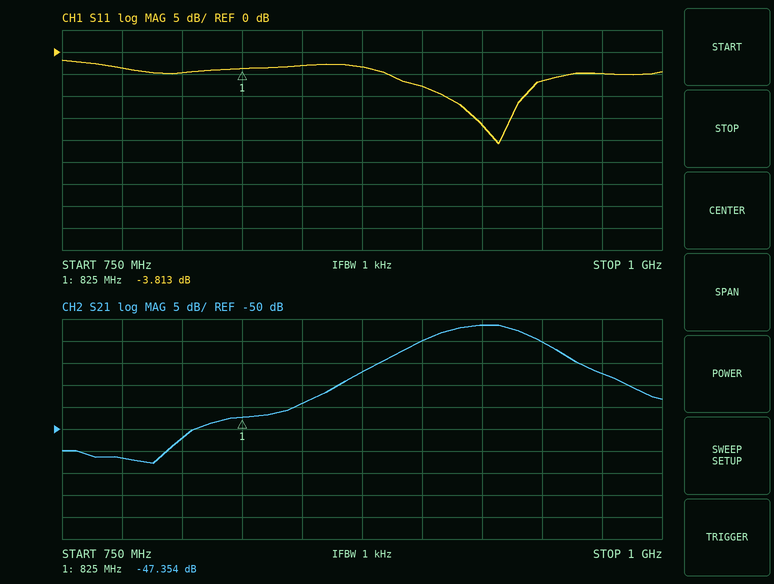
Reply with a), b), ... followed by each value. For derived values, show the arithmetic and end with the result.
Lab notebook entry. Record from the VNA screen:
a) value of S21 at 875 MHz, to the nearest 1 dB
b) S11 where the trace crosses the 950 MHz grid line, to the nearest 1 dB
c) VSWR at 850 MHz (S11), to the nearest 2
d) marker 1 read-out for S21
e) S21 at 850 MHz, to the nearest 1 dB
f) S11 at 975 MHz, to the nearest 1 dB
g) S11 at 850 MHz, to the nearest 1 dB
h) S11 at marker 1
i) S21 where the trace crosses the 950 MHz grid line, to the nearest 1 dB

a) -37 dB
b) -7 dB
c) |Γ| = 10^(-3/20) = 0.7079; VSWR = (1 + 0.7079)/(1 − 0.7079) ≈ 6
d) -47.354 dB
e) -44 dB
f) -5 dB
g) -3 dB
h) -3.813 dB
i) -30 dB
